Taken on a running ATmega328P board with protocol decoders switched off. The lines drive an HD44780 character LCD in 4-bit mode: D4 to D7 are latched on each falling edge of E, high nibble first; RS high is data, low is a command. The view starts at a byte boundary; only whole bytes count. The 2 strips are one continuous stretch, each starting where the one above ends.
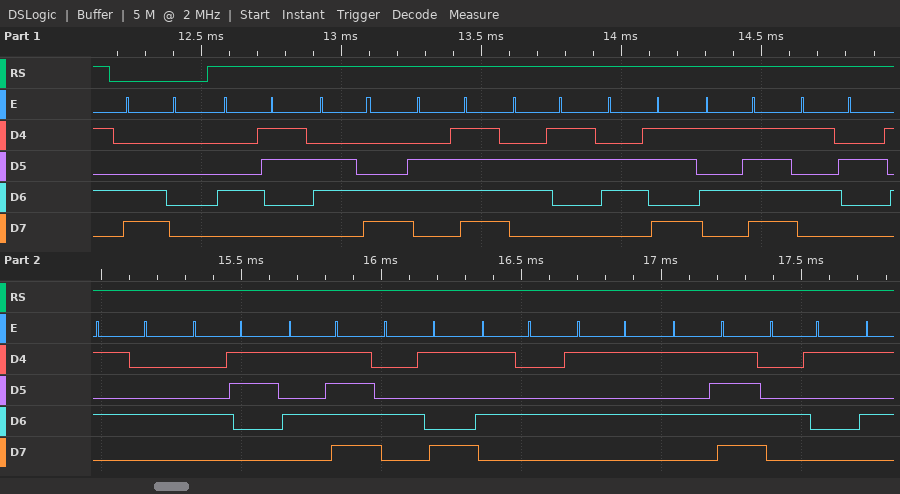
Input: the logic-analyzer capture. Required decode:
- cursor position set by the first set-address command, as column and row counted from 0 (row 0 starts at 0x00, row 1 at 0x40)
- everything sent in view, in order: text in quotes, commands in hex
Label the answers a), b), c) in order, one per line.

a) column 0, row 1
b) 0xC0 "Clock_RTC_ITU_A"
